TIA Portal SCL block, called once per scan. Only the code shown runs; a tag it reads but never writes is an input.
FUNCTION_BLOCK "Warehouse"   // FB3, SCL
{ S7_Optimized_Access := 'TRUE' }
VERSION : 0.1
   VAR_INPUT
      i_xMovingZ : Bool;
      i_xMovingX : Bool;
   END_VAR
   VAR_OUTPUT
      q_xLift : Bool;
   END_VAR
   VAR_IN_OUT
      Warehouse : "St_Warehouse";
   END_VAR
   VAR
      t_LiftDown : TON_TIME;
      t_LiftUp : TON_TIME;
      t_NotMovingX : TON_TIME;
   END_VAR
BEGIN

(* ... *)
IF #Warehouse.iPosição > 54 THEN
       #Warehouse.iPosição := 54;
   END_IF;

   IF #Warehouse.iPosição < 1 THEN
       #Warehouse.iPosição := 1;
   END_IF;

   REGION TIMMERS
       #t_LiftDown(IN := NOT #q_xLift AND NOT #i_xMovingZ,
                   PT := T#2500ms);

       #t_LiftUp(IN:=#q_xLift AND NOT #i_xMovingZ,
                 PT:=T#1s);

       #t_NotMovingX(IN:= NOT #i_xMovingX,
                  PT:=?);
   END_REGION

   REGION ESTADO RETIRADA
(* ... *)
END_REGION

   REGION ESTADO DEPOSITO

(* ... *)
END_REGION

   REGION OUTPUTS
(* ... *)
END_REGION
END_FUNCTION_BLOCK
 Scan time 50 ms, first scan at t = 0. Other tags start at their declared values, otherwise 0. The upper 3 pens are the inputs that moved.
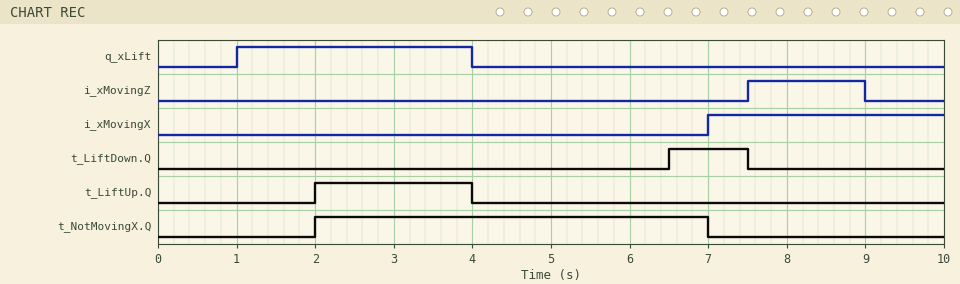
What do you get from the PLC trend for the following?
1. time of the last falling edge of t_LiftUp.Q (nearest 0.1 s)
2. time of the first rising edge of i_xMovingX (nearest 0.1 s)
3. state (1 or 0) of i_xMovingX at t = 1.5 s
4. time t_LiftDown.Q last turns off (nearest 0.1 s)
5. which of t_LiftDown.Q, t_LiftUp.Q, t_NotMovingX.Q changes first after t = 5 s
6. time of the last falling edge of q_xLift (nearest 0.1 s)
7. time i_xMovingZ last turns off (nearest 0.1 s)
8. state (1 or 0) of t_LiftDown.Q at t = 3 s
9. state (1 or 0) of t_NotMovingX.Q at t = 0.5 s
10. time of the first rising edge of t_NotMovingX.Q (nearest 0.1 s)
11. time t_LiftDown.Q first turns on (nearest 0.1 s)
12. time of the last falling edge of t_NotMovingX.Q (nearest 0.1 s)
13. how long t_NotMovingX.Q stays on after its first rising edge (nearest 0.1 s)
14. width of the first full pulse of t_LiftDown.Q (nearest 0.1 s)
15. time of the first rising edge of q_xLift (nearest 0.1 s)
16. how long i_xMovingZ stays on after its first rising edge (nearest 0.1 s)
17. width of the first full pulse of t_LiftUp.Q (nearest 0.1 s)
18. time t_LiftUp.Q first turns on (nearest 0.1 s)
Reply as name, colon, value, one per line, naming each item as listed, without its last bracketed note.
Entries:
time of the last falling edge of t_LiftUp.Q: 4.0 s
time of the first rising edge of i_xMovingX: 7.0 s
state (1 or 0) of i_xMovingX at t = 1.5 s: 0
time t_LiftDown.Q last turns off: 7.5 s
which of t_LiftDown.Q, t_LiftUp.Q, t_NotMovingX.Q changes first after t = 5 s: t_LiftDown.Q
time of the last falling edge of q_xLift: 4.0 s
time i_xMovingZ last turns off: 9.0 s
state (1 or 0) of t_LiftDown.Q at t = 3 s: 0
state (1 or 0) of t_NotMovingX.Q at t = 0.5 s: 0
time of the first rising edge of t_NotMovingX.Q: 2.0 s
time t_LiftDown.Q first turns on: 6.5 s
time of the last falling edge of t_NotMovingX.Q: 7.0 s
how long t_NotMovingX.Q stays on after its first rising edge: 5.0 s
width of the first full pulse of t_LiftDown.Q: 1.0 s
time of the first rising edge of q_xLift: 1.0 s
how long i_xMovingZ stays on after its first rising edge: 1.5 s
width of the first full pulse of t_LiftUp.Q: 2.0 s
time t_LiftUp.Q first turns on: 2.0 s
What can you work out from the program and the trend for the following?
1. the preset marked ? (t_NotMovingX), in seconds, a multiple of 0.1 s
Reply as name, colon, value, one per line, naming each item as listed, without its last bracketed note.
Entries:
the preset marked ? (t_NotMovingX), in seconds, a multiple of 0.1 s: 2.0 s
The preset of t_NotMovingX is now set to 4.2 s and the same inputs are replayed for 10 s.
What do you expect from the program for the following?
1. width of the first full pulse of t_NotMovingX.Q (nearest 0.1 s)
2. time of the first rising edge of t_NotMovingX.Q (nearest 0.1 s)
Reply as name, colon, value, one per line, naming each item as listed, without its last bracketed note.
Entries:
width of the first full pulse of t_NotMovingX.Q: 2.8 s
time of the first rising edge of t_NotMovingX.Q: 4.2 s
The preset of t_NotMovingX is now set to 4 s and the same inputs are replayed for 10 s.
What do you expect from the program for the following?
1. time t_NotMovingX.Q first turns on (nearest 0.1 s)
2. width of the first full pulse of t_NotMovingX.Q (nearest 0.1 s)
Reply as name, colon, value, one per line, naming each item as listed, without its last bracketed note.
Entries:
time t_NotMovingX.Q first turns on: 4.0 s
width of the first full pulse of t_NotMovingX.Q: 3.0 s
